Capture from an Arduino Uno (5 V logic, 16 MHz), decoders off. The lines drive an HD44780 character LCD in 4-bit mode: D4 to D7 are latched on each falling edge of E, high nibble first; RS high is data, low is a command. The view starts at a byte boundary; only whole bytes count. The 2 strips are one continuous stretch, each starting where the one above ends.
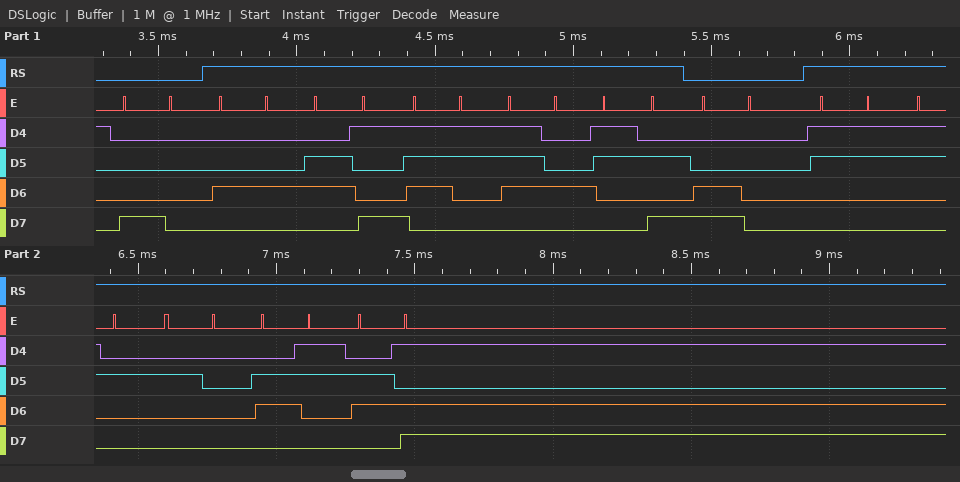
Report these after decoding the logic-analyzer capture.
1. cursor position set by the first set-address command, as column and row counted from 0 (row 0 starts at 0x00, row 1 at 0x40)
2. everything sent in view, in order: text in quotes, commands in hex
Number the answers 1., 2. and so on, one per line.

1. column 0, row 0
2. 0x80 "Dist:" 0xC0 "32 cm"
